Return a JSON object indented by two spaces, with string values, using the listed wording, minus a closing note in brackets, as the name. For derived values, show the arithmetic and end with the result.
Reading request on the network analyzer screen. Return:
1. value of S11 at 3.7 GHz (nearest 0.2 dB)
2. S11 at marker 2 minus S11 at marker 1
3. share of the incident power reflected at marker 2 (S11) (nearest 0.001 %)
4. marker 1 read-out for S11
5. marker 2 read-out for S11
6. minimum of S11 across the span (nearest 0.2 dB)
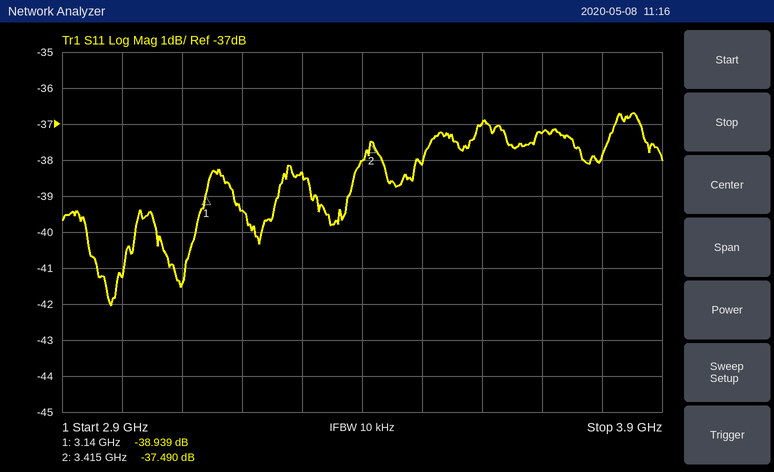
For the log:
{
  "value of S11 at 3.7 GHz": "-37.2 dB",
  "S11 at marker 2 minus S11 at marker 1": "-37.49 − (-38.939) = 1.449 dB",
  "share of the incident power reflected at marker 2 (S11)": "10^(-37.49/10) ≈ 0.018 %",
  "marker 1 read-out for S11": "-38.939 dB",
  "marker 2 read-out for S11": "-37.490 dB",
  "minimum of S11 across the span": "-42.0 dB"
}
